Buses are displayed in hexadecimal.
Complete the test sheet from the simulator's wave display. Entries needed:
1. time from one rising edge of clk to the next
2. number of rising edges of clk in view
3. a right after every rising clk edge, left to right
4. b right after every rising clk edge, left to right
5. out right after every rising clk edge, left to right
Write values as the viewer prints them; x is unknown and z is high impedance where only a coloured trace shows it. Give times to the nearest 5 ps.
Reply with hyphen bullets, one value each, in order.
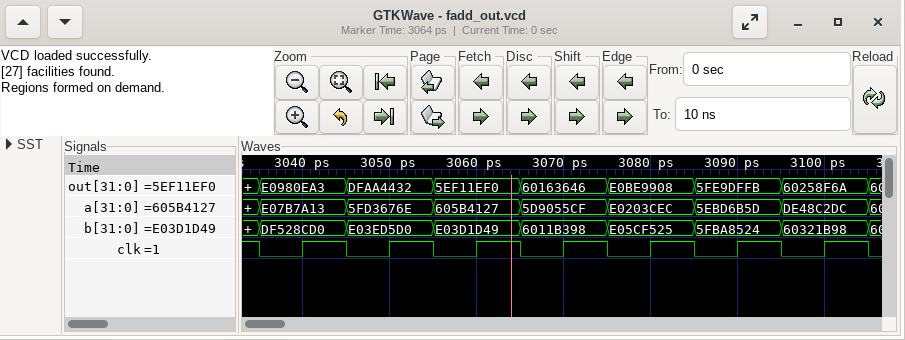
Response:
- 10 ps
- 7
- E07B7A13, 5FD3676E, 605B4127, 5D9055CF, E0203CEC, 5EBD6B5D, DE48C2DC
- DF528CD0, E03ED5D0, E03D1D49, 6011B398, E05CF525, 5FBA8524, 60321B98
- E0980EA3, DFAA4432, 5EF11EF0, 60163646, E0BE9908, 5FE9DFFB, 60258F6A
